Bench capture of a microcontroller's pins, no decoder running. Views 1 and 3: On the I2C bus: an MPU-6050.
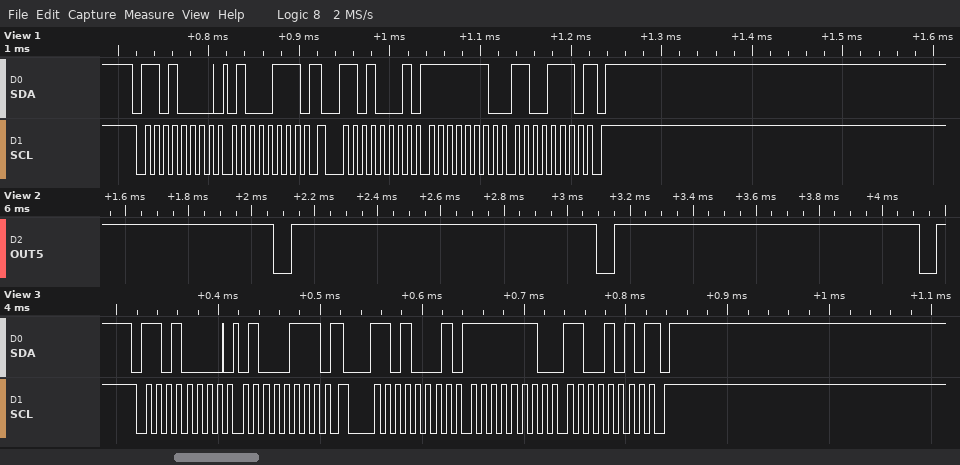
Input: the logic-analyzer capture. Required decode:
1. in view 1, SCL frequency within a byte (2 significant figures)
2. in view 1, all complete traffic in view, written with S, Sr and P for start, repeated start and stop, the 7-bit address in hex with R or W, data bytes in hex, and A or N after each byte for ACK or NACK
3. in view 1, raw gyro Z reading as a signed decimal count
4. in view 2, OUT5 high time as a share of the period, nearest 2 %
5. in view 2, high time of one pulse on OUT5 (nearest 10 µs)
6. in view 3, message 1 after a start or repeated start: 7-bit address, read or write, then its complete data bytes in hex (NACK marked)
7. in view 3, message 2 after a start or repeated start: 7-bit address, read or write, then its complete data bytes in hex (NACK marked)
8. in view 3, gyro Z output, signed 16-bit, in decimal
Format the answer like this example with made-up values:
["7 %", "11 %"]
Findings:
["100 kHz", "S 68W A 47 A Sr 68R A FE A CE N P", "-306", "94 %", "970 µs", "0x68 write: 47", "0x68 read: FE CA NACK", "-310"]
